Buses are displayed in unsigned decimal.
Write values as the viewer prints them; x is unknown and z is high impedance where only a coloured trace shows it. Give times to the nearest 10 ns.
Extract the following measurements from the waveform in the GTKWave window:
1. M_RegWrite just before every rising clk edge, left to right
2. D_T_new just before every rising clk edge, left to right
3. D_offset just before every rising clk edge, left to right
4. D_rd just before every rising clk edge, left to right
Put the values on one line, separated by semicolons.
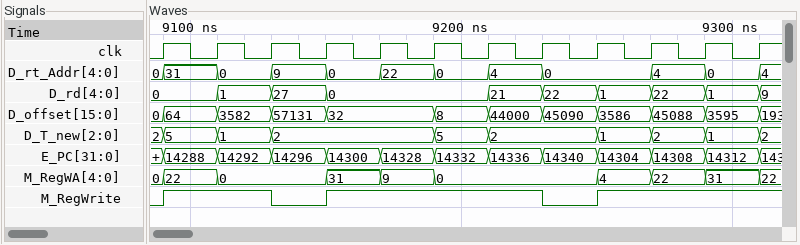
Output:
0 1 1 0 1 1 1 1 0 1 1 1; 2, 5, 1, 2, 2, 2, 5, 2, 2, 1, 2, 1; 0, 64, 3582, 57131, 32, 32, 8, 44000, 45090, 3586, 45088, 3595; 0, 0, 1, 27, 0, 0, 0, 21, 22, 1, 22, 1
